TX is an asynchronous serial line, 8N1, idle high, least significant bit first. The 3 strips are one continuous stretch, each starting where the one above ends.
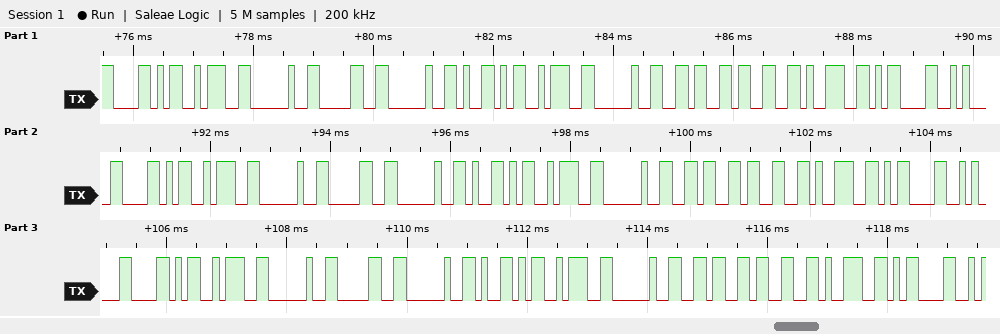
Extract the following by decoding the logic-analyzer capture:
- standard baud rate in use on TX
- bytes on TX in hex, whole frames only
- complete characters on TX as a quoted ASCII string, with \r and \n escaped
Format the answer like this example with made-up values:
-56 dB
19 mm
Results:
9600 baud
0x58 0x3A 0x20 0x30 0x20 0x59 0x3A 0x20 0x36 0x33 0x39 0x0D 0x0A 0x58 0x3A 0x20 0x30 0x20 0x59 0x3A 0x20 0x36 0x33 0x39 0x0D 0x0A 0x58 0x3A 0x20 0x30 0x20 0x59 0x3A 0x20 0x36 0x33 0x39 0x0D
"X: 0 Y: 639\r\nX: 0 Y: 639\r\nX: 0 Y: 639\r"
